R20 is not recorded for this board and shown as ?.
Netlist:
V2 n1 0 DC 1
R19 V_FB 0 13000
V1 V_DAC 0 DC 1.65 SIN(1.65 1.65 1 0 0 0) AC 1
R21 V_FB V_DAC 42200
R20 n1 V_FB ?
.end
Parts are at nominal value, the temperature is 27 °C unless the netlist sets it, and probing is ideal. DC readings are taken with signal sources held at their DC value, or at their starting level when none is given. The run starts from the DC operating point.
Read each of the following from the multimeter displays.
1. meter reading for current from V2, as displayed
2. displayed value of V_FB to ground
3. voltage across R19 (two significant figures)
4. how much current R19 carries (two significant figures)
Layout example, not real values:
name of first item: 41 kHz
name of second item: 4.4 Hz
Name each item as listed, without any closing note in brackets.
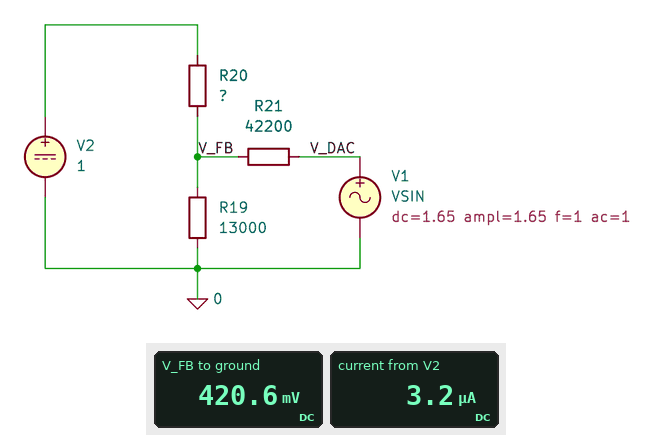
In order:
meter reading for current from V2, as displayed: 3.2 µA
displayed value of V_FB to ground: 420.6 mV
voltage across R19: 420 mV
how much current R19 carries: 32 µA
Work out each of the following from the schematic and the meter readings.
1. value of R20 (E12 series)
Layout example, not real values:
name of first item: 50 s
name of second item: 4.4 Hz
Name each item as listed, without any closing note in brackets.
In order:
value of R20: 180 kΩ
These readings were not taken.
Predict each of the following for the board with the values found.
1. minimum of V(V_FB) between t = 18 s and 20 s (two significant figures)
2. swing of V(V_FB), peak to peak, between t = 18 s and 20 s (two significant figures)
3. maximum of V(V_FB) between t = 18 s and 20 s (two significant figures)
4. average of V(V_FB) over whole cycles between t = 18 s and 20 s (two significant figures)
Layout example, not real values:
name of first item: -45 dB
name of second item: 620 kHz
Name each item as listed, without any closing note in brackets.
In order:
minimum of V(V_FB) between t = 18 s and 20 s: 52 mV
swing of V(V_FB), peak to peak, between t = 18 s and 20 s: 740 mV
maximum of V(V_FB) between t = 18 s and 20 s: 790 mV
average of V(V_FB) over whole cycles between t = 18 s and 20 s: 420 mV
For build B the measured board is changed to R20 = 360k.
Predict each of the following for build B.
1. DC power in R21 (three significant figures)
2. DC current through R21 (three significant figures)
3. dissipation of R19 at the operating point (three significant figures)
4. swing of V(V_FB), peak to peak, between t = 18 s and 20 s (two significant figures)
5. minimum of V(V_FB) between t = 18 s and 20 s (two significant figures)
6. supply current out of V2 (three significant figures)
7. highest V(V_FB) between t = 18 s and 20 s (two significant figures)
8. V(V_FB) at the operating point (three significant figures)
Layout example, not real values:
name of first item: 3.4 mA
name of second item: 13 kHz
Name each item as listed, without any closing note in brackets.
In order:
DC power in R21: 36.7 µW
DC current through R21: 29.5 µA
dissipation of R19 at the operating point: 12.6 µW
swing of V(V_FB), peak to peak, between t = 18 s and 20 s: 760 mV
minimum of V(V_FB) between t = 18 s and 20 s: 27 mV
supply current out of V2: 1.65 µA
highest V(V_FB) between t = 18 s and 20 s: 780 mV
V(V_FB) at the operating point: 405 mV
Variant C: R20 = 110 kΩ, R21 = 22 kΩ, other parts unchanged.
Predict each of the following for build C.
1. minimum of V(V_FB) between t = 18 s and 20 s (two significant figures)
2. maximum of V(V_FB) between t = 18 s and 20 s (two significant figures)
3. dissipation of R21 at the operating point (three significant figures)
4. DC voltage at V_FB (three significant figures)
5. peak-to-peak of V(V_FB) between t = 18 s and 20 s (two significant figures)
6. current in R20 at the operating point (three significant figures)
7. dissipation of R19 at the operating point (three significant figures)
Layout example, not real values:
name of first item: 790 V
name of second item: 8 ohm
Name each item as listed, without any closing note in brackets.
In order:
minimum of V(V_FB) between t = 18 s and 20 s: 69 mV
maximum of V(V_FB) between t = 18 s and 20 s: 1.2 V
dissipation of R21 at the operating point: 46.4 µW
DC voltage at V_FB: 640 mV
peak-to-peak of V(V_FB) between t = 18 s and 20 s: 1.1 V
current in R20 at the operating point: 3.28 µA
dissipation of R19 at the operating point: 31.5 µW
